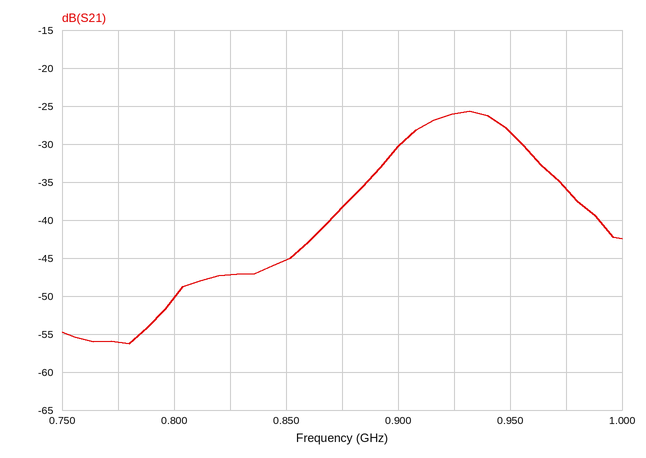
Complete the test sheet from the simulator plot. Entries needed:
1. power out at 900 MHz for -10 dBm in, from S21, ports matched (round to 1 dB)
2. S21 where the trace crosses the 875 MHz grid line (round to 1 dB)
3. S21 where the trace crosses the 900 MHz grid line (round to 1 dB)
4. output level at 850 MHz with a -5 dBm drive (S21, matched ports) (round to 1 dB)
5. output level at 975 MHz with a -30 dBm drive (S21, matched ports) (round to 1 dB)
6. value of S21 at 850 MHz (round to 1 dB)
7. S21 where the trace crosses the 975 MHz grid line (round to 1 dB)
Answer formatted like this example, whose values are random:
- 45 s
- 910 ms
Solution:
- -40 dBm
- -38 dB
- -30 dB
- -50 dBm
- -66 dBm
- -45 dB
- -36 dB
